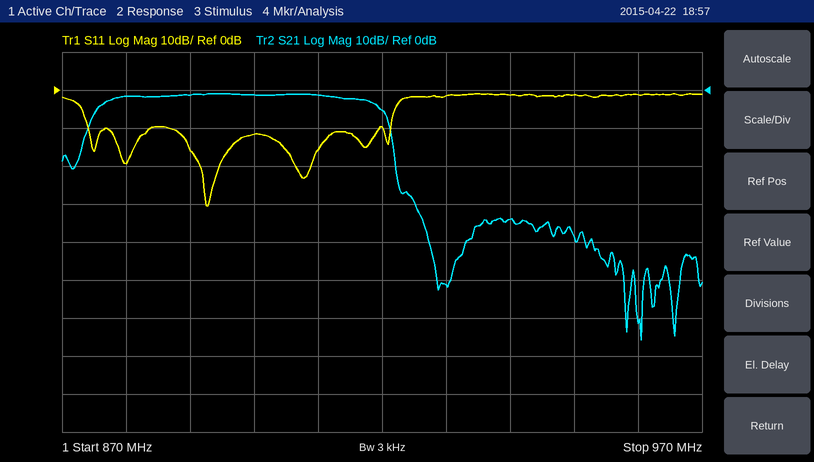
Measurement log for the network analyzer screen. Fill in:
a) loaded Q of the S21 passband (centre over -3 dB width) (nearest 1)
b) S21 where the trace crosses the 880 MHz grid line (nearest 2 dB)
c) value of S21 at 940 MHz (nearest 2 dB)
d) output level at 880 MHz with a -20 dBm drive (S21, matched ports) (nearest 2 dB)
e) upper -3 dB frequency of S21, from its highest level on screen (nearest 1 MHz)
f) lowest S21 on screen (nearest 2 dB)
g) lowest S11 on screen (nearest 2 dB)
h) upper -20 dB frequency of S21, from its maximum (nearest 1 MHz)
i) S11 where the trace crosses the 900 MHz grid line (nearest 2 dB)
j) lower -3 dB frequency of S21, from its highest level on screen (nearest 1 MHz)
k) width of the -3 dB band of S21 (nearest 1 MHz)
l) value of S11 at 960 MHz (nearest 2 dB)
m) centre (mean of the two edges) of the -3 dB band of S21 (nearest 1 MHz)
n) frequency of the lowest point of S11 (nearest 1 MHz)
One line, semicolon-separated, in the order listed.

21; -2 dB; -34 dB; -22 dBm; 919 MHz; -66 dB; -30 dB; 922 MHz; -12 dB; 876 MHz; 43 MHz; -2 dB; 898 MHz; 893 MHz
